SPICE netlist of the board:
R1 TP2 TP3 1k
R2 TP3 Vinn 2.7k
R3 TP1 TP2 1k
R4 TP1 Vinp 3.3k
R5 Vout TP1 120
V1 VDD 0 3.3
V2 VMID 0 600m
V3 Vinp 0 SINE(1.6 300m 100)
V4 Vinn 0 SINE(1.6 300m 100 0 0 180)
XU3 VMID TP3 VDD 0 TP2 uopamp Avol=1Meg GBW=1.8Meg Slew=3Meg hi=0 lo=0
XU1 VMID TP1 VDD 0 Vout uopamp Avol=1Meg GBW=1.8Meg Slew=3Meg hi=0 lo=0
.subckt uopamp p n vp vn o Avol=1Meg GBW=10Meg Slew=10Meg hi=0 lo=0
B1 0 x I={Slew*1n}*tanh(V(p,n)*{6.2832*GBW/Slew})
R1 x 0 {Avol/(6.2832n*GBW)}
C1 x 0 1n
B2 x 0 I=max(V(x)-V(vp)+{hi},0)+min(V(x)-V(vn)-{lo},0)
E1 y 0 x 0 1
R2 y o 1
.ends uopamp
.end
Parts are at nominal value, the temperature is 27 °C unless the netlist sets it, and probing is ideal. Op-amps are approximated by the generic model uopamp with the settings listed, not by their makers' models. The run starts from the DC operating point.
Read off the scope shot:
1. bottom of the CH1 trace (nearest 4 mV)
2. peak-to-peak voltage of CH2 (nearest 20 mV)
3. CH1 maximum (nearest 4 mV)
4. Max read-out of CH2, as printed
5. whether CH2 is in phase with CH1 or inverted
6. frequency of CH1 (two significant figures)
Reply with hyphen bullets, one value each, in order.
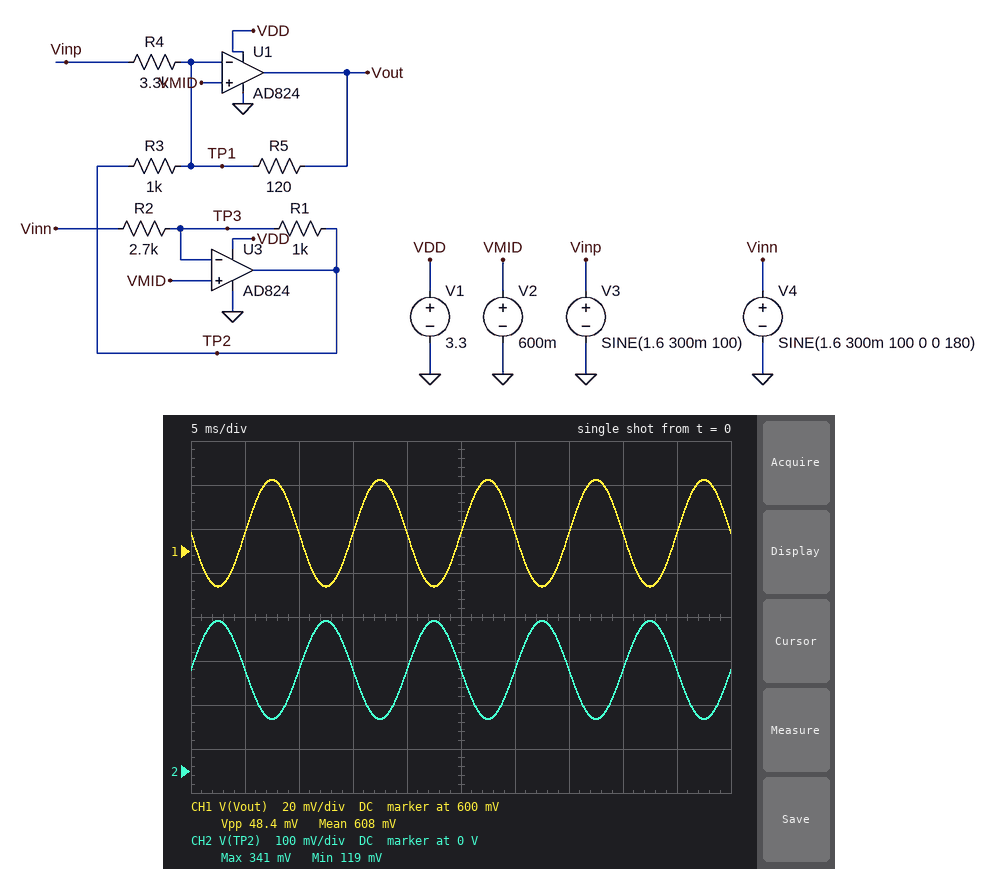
- 584 mV
- 220 mV
- 632 mV
- 341 mV
- inverted
- 100 Hz
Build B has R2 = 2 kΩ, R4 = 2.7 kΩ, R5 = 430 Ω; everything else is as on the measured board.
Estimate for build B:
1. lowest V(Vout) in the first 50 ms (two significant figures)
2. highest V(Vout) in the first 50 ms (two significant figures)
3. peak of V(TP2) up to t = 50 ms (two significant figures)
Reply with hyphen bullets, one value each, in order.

- 540 mV
- 750 mV
- 250 mV
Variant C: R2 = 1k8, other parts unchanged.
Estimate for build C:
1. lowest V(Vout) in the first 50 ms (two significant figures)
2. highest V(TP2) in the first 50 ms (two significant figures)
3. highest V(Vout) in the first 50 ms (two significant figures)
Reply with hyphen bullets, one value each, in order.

- 600 mV
- 210 mV
- 650 mV
